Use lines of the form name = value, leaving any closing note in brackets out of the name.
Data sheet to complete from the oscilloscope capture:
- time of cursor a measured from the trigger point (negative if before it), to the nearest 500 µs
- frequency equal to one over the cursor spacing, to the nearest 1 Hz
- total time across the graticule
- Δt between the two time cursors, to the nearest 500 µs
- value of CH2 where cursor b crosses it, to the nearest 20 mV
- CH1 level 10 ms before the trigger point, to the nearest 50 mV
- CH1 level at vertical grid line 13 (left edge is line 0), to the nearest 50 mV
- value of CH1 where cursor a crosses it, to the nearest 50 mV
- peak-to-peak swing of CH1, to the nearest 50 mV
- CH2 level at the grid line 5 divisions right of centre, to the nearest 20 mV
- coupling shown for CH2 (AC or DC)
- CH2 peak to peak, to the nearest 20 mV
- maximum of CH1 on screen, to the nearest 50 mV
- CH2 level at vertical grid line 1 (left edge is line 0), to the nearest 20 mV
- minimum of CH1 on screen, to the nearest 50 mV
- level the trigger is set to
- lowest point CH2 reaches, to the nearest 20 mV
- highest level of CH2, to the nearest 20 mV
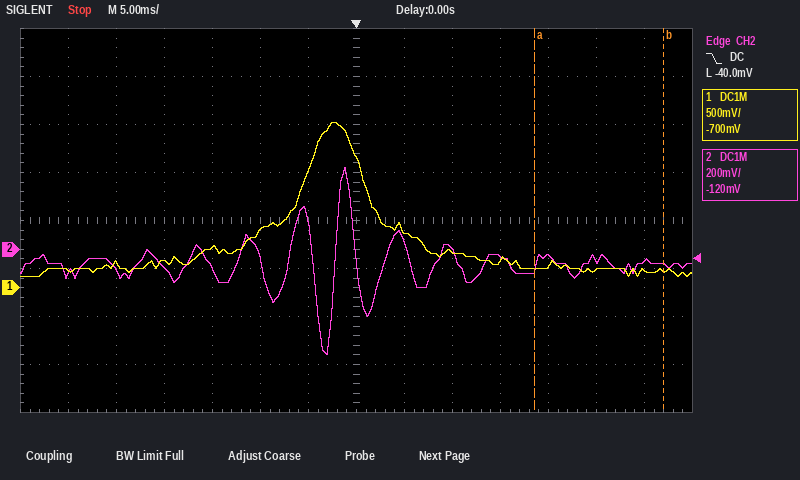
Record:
time of cursor a measured from the trigger point (negative if before it), to the nearest 500 µs = +18.5 ms
frequency equal to one over the cursor spacing, to the nearest 1 Hz = 74 Hz
total time across the graticule = 70 ms
Δt between the two time cursors, to the nearest 500 µs = 13.5 ms
value of CH2 where cursor b crosses it, to the nearest 20 mV = -60 mV
CH1 level 10 ms before the trigger point, to the nearest 50 mV = 600 mV
CH1 level at vertical grid line 13 (left edge is line 0), to the nearest 50 mV = 200 mV
value of CH1 where cursor a crosses it, to the nearest 50 mV = 200 mV
peak-to-peak swing of CH1, to the nearest 50 mV = 1.60 V
CH2 level at the grid line 5 divisions right of centre, to the nearest 20 mV = -40 mV
coupling shown for CH2 = DC
CH2 peak to peak, to the nearest 20 mV = 780 mV
maximum of CH1 on screen, to the nearest 50 mV = 1.70 V
CH2 level at vertical grid line 1 (left edge is line 0), to the nearest 20 mV = -100 mV
minimum of CH1 on screen, to the nearest 50 mV = 100 mV
level the trigger is set to = -40.0 mV
lowest point CH2 reaches, to the nearest 20 mV = -440 mV
highest level of CH2, to the nearest 20 mV = 340 mV
